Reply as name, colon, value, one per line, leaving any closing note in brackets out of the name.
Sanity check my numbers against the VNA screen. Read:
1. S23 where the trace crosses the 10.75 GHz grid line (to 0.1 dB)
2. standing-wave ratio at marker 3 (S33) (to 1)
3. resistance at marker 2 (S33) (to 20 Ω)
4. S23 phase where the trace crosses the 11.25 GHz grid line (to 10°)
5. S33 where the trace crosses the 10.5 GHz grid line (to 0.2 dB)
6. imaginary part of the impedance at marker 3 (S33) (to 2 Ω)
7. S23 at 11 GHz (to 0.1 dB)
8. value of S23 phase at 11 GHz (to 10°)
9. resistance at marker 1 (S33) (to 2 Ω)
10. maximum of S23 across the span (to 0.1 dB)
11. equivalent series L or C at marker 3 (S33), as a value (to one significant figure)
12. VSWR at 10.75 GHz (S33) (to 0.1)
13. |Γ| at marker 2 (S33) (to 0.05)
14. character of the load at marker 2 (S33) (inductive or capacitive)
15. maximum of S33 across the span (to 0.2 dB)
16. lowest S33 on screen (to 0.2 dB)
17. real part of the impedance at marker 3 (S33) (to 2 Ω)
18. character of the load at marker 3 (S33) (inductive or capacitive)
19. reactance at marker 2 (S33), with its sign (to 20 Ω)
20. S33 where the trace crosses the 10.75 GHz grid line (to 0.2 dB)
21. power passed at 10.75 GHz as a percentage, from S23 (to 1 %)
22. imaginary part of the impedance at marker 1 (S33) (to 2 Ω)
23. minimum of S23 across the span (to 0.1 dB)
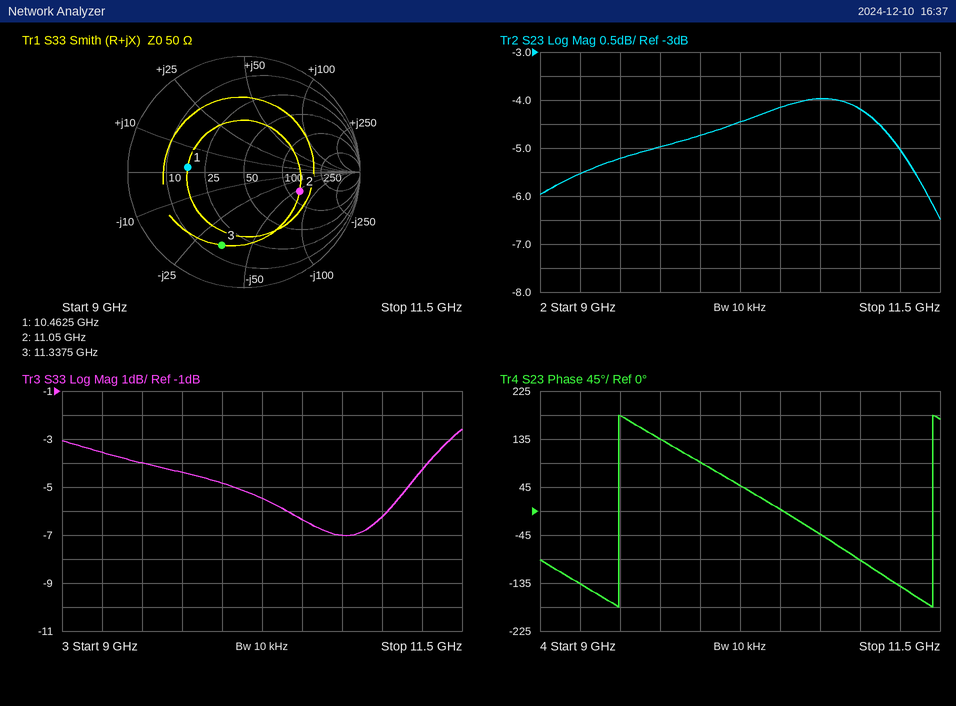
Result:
S23 where the trace crosses the 10.75 GHz grid line: -4.0 dB
standing-wave ratio at marker 3 (S33): 5
resistance at marker 2 (S33): 120 Ω
S23 phase where the trace crosses the 11.25 GHz grid line: -140°
S33 where the trace crosses the 10.5 GHz grid line: -6.4 dB
imaginary part of the impedance at marker 3 (S33): -34 Ω
S23 at 11 GHz: -4.2 dB
value of S23 phase at 11 GHz: -90°
resistance at marker 1 (S33): 18 Ω
maximum of S23 across the span: -4.0 dB
equivalent series L or C at marker 3 (S33), as a value: 400 fF
VSWR at 10.75 GHz (S33): 2.6
|Γ| at marker 2 (S33): 0.50
character of the load at marker 2 (S33): capacitive
maximum of S33 across the span: -2.6 dB
lowest S33 on screen: -7.0 dB
real part of the impedance at marker 3 (S33): 16 Ω
character of the load at marker 3 (S33): capacitive
reactance at marker 2 (S33), with its sign: -60 Ω
S33 where the trace crosses the 10.75 GHz grid line: -7.0 dB
power passed at 10.75 GHz as a percentage, from S23: 40 %
imaginary part of the impedance at marker 1 (S33): +2 Ω
minimum of S23 across the span: -6.5 dB
